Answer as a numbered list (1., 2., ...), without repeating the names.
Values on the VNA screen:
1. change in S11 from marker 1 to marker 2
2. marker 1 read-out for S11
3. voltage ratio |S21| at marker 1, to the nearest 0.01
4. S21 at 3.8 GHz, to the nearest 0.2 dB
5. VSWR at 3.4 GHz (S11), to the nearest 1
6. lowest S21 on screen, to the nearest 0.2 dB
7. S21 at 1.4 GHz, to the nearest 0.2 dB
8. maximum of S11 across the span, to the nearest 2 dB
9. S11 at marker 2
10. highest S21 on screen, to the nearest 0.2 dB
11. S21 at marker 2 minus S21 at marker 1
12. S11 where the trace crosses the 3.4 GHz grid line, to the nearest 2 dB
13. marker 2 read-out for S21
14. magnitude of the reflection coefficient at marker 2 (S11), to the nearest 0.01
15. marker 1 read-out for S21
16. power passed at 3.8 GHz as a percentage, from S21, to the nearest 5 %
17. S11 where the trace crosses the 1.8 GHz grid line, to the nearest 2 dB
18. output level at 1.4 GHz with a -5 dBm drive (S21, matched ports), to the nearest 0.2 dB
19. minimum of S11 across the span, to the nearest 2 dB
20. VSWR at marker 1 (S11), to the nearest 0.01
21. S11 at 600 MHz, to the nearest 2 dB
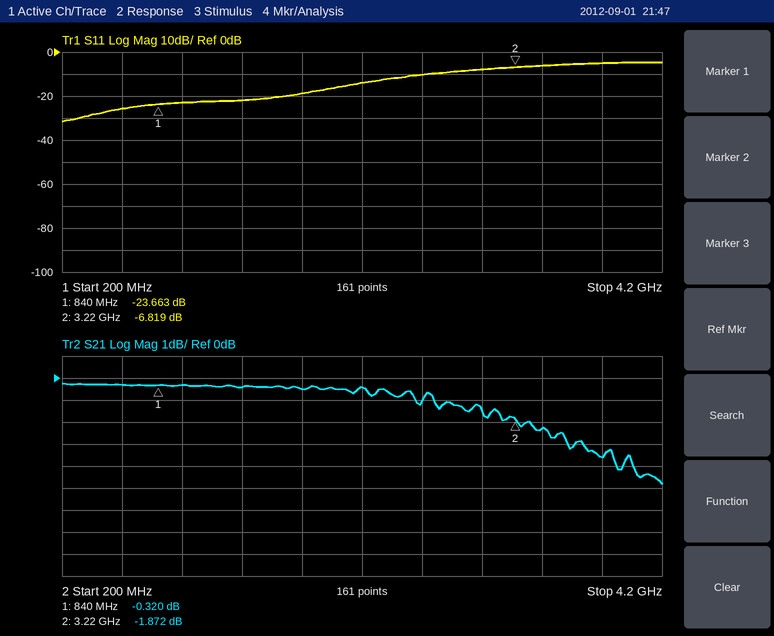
1. 16.844 dB
2. -23.663 dB
3. 0.96
4. -3.6 dB
5. 3
6. -4.8 dB
7. -0.4 dB
8. -4 dB
9. -6.819 dB
10. -0.2 dB
11. -1.552 dB
12. -6 dB
13. -1.872 dB
14. 0.46
15. -0.320 dB
16. 45 %
17. -18 dB
18. -5.4 dBm
19. -32 dB
20. 1.14
21. -26 dB
